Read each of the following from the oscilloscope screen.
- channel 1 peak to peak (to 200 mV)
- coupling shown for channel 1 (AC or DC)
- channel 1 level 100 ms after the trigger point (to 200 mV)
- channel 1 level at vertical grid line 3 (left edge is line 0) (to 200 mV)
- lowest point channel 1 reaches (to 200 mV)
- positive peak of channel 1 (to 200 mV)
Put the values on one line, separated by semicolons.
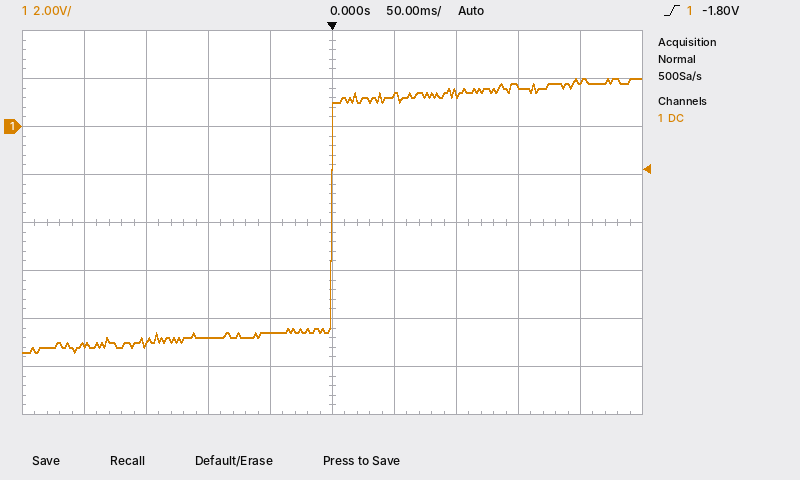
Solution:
11.4 V; DC; 1.4 V; -8.8 V; -9.4 V; 2.0 V
